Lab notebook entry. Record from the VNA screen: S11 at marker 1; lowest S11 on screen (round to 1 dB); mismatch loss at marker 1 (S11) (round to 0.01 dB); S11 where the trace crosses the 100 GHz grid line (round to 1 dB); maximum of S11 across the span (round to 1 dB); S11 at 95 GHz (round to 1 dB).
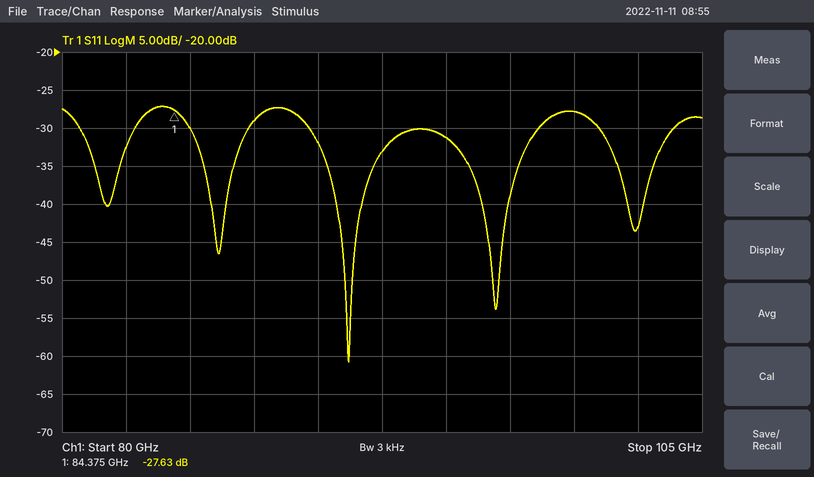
-27.63 dB
-61 dB
0.01 dB
-28 dB
-27 dB
-31 dB
